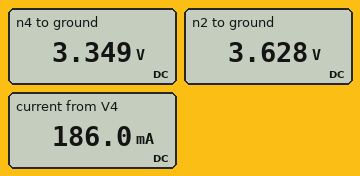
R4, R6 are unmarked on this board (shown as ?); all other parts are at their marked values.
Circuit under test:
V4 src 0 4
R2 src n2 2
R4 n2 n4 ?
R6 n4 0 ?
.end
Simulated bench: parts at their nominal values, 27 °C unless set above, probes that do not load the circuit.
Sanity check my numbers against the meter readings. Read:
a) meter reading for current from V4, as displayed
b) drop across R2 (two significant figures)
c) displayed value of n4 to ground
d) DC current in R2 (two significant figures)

186.0 mA
370 mV
3.349 V
190 mA
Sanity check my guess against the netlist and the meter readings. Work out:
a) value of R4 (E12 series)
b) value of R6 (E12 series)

1.5 Ω
18 Ω
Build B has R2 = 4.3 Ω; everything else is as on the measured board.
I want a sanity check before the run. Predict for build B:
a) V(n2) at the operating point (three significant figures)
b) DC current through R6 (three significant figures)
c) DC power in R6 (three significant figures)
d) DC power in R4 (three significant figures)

3.28 V
168 mA
508 mW
42.4 mW
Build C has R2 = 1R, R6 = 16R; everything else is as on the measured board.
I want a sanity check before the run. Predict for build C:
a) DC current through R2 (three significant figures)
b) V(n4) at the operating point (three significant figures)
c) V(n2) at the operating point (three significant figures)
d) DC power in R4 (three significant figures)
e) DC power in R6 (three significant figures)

216 mA
3.46 V
3.78 V
70.1 mW
748 mW
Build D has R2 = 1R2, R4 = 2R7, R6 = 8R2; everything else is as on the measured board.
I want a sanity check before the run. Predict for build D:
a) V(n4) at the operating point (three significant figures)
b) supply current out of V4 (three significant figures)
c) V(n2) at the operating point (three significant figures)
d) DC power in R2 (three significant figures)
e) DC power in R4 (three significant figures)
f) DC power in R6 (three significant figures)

2.71 V
331 mA
3.60 V
131 mW
295 mW
896 mW
